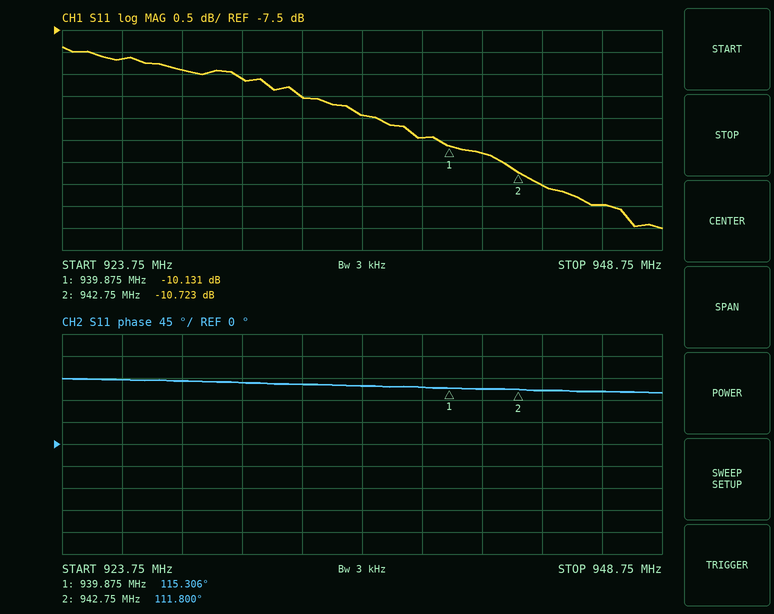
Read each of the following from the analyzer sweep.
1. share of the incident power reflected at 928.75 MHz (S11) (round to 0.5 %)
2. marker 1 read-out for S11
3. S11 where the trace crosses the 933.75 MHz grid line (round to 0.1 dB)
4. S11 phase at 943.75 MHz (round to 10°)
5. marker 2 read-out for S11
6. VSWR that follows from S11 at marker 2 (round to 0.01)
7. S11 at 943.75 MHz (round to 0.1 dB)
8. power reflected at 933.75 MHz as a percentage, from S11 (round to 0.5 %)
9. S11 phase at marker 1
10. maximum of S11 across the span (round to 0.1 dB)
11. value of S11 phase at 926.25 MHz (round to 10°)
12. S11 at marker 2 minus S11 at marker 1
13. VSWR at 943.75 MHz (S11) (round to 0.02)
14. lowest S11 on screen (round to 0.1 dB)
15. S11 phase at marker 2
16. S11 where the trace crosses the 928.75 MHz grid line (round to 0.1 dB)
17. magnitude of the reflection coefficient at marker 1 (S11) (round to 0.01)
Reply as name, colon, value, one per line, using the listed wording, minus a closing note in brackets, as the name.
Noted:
share of the incident power reflected at 928.75 MHz (S11): 14.5 %
marker 1 read-out for S11: -10.131 dB
S11 where the trace crosses the 933.75 MHz grid line: -9.0 dB
S11 phase at 943.75 MHz: 110°
marker 2 read-out for S11: -10.723 dB
VSWR that follows from S11 at marker 2: 1.82
S11 at 943.75 MHz: -11.0 dB
power reflected at 933.75 MHz as a percentage, from S11: 12.5 %
S11 phase at marker 1: 115.306°
maximum of S11 across the span: -7.9 dB
value of S11 phase at 926.25 MHz: 130°
S11 at marker 2 minus S11 at marker 1: -0.592 dB
VSWR at 943.75 MHz (S11): 1.78
lowest S11 on screen: -12.0 dB
S11 phase at marker 2: 111.800°
S11 where the trace crosses the 928.75 MHz grid line: -8.4 dB
magnitude of the reflection coefficient at marker 1 (S11): 0.31
